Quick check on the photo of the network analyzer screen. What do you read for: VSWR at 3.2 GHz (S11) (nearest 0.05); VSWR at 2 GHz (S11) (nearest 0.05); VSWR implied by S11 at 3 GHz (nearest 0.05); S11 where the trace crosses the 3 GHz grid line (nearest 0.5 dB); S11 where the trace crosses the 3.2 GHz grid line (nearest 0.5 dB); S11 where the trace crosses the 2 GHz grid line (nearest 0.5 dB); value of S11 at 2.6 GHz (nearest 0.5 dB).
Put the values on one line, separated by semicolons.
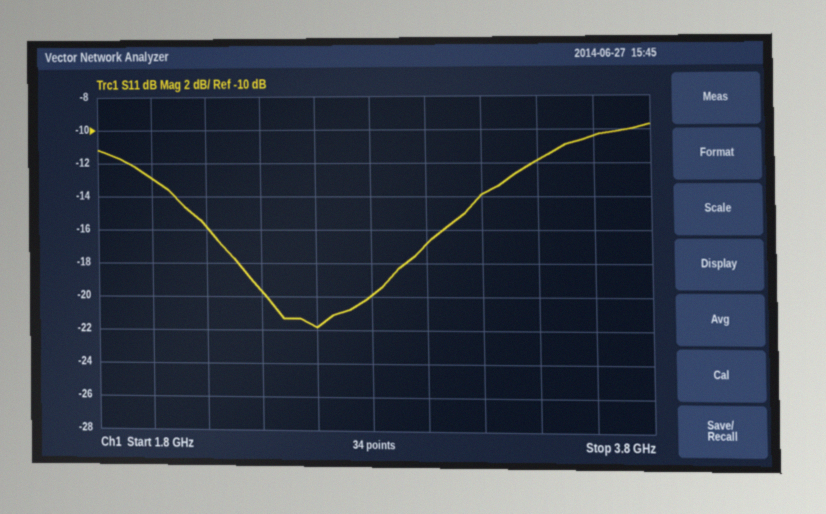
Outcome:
1.50; 1.60; 1.35; -17.0 dB; -14.0 dB; -13.0 dB; -22.0 dB
